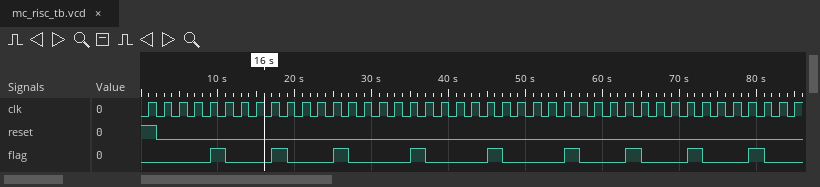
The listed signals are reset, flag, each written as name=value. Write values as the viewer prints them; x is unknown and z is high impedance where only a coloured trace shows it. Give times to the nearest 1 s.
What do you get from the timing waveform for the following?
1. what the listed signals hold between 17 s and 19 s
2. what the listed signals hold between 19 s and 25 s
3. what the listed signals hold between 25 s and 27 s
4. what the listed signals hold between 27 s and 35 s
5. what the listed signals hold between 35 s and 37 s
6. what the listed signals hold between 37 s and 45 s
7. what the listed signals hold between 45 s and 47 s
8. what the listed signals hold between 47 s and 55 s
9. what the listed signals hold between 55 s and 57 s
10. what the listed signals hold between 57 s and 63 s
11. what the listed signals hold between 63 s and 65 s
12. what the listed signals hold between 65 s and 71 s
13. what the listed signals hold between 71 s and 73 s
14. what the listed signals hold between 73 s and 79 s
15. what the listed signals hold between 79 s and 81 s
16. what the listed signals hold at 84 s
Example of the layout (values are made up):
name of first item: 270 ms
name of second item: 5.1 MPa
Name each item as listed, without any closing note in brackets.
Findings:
what the listed signals hold between 17 s and 19 s: reset=0, flag=1
what the listed signals hold between 19 s and 25 s: reset=0, flag=0
what the listed signals hold between 25 s and 27 s: reset=0, flag=1
what the listed signals hold between 27 s and 35 s: reset=0, flag=0
what the listed signals hold between 35 s and 37 s: reset=0, flag=1
what the listed signals hold between 37 s and 45 s: reset=0, flag=0
what the listed signals hold between 45 s and 47 s: reset=0, flag=1
what the listed signals hold between 47 s and 55 s: reset=0, flag=0
what the listed signals hold between 55 s and 57 s: reset=0, flag=1
what the listed signals hold between 57 s and 63 s: reset=0, flag=0
what the listed signals hold between 63 s and 65 s: reset=0, flag=1
what the listed signals hold between 65 s and 71 s: reset=0, flag=0
what the listed signals hold between 71 s and 73 s: reset=0, flag=1
what the listed signals hold between 73 s and 79 s: reset=0, flag=0
what the listed signals hold between 79 s and 81 s: reset=0, flag=1
what the listed signals hold at 84 s: reset=0, flag=0
